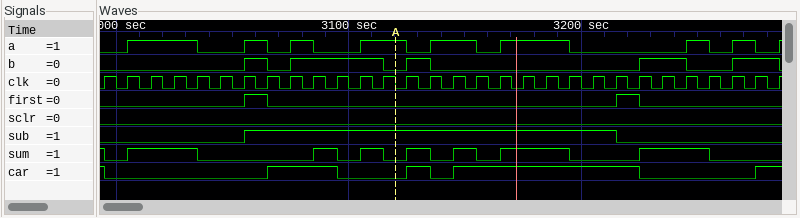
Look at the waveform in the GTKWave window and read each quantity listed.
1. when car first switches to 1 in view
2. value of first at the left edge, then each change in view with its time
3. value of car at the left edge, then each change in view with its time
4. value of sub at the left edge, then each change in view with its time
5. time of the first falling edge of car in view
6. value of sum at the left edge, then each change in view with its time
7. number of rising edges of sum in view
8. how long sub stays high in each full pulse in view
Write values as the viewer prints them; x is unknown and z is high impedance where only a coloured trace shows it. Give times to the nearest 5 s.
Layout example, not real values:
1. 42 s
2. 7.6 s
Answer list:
1. 3065 s
2. 0, 1 at 3055 s, 0 at 3065 s, 1 at 3215 s, 0 at 3225 s
3. 1, 0 at 2995 s, 1 at 3065 s, 0 at 3095 s, 1 at 3125 s, 0 at 3135 s, 1 at 3145 s, 0 at 3225 s, 1 at 3275 s
4. 0, 1 at 3055 s, 0 at 3215 s
5. 2995 s
6. 1, 0 at 2995 s, 1 at 3005 s, 0 at 3035 s, 1 at 3085 s, 0 at 3095 s, 1 at 3105 s, 0 at 3115 s, 1 at 3125 s, 0 at 3135 s, 1 at 3145 s, 0 at 3155 s, 1 at 3165 s, 0 at 3195 s, 1 at 3225 s, 0 at 3255 s
7. 7
8. 160 s
